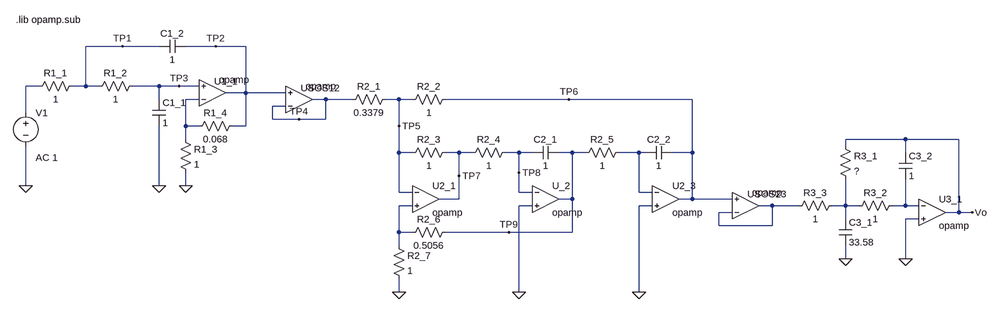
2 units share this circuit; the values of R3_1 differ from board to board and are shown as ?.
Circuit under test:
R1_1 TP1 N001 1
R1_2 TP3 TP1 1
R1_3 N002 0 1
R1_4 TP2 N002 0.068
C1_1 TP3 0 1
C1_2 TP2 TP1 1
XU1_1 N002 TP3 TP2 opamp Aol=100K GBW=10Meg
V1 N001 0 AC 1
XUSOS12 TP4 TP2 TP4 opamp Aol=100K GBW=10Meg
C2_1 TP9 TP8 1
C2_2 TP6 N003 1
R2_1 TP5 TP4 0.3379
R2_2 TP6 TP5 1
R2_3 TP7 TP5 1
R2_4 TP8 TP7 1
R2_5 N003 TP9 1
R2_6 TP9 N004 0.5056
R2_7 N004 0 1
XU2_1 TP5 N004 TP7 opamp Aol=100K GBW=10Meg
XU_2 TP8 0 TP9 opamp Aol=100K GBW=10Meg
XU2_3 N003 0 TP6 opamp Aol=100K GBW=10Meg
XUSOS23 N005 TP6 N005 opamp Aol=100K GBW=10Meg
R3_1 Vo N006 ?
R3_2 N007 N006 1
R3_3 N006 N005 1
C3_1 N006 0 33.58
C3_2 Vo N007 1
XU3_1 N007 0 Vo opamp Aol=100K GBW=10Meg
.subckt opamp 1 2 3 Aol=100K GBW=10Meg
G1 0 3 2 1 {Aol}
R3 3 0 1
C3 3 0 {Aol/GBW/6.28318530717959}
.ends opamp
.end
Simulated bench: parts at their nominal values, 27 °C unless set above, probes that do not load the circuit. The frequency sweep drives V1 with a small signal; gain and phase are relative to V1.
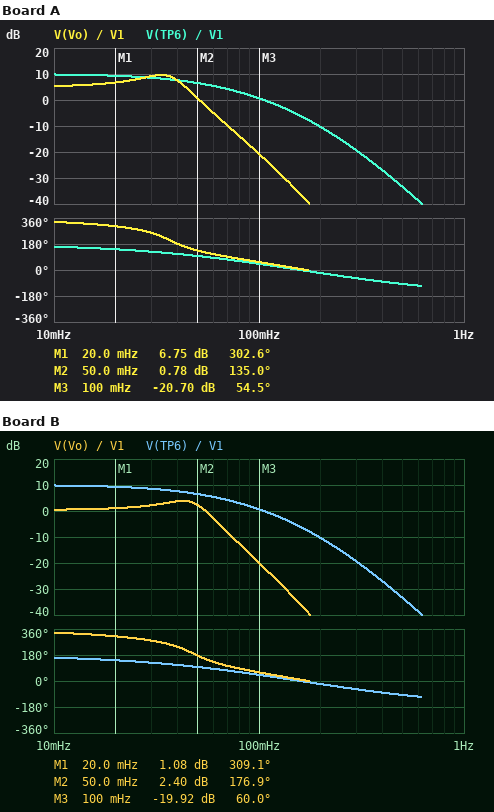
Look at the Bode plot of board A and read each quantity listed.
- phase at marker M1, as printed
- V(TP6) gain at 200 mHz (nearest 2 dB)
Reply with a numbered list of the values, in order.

1. 302.6 deg
2. -10 dB
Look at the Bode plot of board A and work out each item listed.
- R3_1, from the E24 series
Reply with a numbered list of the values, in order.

1. 0.56 Ω
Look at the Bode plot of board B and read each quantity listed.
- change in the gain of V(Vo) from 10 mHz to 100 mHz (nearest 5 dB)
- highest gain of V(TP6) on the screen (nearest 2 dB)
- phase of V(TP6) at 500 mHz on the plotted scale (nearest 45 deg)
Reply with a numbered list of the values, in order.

1. -20 dB
2. 10 dB
3. -90 deg
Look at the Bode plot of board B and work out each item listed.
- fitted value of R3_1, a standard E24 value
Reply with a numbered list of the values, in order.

1. 0.33 Ω
